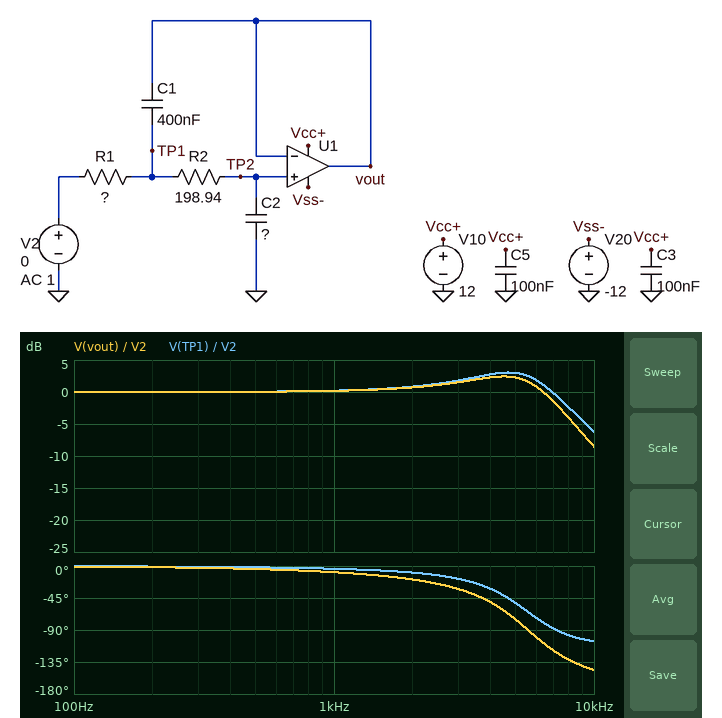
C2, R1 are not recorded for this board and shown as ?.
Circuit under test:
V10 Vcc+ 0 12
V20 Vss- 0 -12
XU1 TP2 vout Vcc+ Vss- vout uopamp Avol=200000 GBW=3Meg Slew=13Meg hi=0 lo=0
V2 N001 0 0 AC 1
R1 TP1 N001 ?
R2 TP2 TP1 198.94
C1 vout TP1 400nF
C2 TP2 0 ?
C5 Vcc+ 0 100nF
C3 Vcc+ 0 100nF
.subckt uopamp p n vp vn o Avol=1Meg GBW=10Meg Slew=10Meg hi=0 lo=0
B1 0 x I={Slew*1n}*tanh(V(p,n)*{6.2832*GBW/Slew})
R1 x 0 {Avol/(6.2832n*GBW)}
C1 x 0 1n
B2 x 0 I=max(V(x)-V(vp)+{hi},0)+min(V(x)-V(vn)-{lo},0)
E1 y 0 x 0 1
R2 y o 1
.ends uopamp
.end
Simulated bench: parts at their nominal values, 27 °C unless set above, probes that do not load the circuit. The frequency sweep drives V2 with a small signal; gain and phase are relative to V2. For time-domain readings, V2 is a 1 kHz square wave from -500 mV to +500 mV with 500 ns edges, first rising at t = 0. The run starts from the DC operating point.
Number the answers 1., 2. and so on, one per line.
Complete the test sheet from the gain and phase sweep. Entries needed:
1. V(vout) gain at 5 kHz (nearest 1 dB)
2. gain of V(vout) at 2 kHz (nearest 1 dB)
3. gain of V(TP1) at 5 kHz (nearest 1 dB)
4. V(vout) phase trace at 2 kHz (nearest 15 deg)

1. 2 dB
2. 1 dB
3. 3 dB
4. -15 deg
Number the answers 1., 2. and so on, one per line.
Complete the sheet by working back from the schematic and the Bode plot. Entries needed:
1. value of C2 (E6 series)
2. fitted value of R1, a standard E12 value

1. 68 nF
2. 150 Ω
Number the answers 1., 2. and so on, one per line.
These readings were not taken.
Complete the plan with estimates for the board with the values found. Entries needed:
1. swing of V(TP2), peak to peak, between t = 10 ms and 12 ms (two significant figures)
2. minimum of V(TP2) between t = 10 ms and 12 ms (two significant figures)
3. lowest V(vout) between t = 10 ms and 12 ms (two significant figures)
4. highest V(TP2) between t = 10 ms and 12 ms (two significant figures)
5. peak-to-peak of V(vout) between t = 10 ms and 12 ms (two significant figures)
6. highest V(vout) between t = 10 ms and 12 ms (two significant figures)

1. 1.5 V
2. -740 mV
3. -740 mV
4. 740 mV
5. 1.5 V
6. 740 mV
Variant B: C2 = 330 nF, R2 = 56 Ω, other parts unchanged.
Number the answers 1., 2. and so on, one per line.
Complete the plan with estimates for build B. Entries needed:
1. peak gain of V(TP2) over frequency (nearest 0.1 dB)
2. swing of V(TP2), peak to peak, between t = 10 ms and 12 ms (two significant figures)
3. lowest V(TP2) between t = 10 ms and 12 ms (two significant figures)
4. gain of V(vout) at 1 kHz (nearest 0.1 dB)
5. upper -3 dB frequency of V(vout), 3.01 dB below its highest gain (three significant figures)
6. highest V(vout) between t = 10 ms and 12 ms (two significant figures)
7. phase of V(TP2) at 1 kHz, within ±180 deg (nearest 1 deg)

1. 0 dB
2. 1.0 V
3. -500 mV
4. -0.4 dB
5. 2.99 kHz
6. 500 mV
7. -24 deg
